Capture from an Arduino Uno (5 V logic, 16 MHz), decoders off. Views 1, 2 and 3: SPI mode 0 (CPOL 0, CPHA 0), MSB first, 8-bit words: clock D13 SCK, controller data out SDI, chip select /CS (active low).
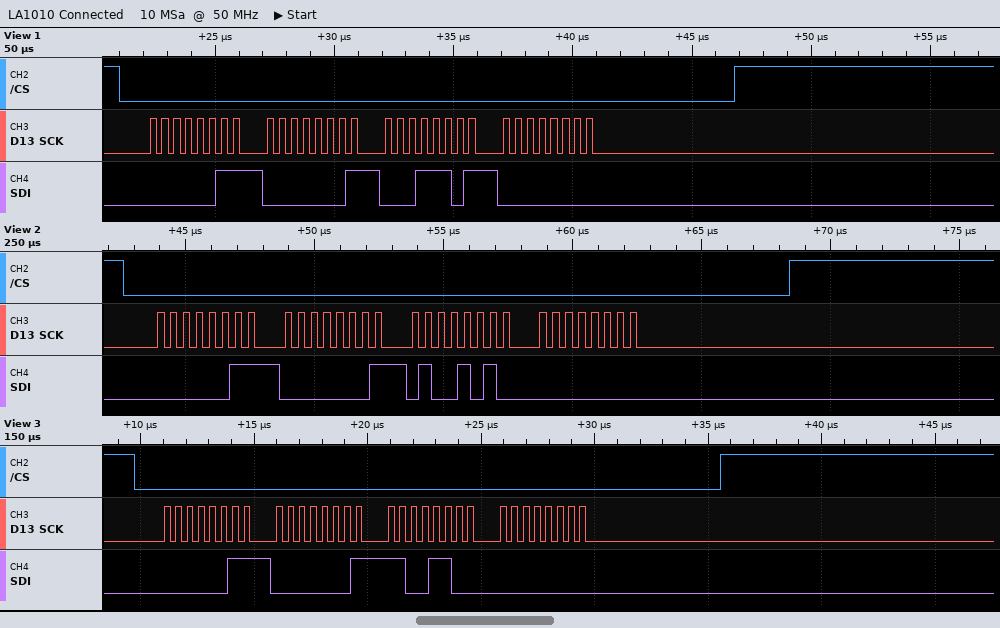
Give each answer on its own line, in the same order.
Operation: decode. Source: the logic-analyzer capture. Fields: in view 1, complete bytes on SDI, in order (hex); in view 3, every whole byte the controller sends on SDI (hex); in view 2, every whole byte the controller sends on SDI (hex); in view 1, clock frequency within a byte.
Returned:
03 01 1D 00
03 01 CC 00
03 01 4A 00
2 MHz
